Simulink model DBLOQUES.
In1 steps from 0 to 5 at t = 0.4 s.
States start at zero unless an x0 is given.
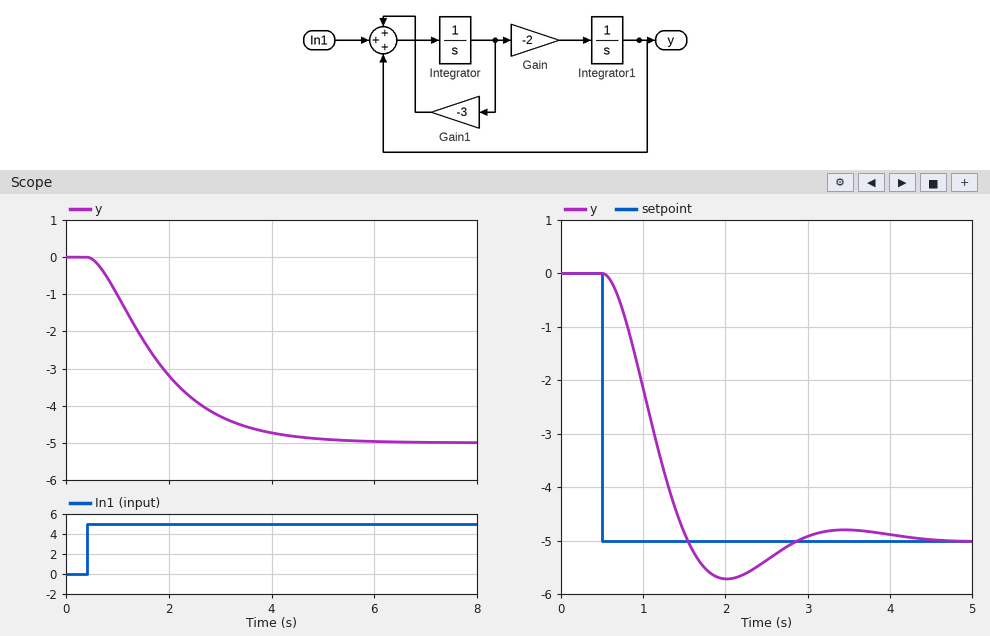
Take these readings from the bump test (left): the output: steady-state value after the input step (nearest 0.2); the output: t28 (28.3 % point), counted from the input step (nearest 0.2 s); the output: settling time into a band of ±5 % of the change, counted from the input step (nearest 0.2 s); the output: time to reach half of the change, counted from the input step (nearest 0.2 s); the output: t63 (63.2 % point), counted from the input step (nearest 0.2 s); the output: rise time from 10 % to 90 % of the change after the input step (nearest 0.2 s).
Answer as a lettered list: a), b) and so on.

a) -5.0
b) 0.8 s
c) 3.6 s
d) 1.2 s
e) 1.6 s
f) 2.6 s
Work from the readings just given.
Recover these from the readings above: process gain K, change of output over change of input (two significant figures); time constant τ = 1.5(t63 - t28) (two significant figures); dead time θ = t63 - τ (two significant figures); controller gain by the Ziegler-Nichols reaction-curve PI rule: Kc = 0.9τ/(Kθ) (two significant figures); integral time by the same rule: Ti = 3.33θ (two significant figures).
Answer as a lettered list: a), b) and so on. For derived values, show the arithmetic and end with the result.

a) (-5 - 0) / 5 = -1.0
b) 1.5 × (1.6 - 0.8) = 1.2 s
c) 1.6 - 1.2 = 0.40 s
d) 0.9 × 1.2 / (-1 × 0.4) = -2.7
e) 3.33 × 0.4 = 1.3 s
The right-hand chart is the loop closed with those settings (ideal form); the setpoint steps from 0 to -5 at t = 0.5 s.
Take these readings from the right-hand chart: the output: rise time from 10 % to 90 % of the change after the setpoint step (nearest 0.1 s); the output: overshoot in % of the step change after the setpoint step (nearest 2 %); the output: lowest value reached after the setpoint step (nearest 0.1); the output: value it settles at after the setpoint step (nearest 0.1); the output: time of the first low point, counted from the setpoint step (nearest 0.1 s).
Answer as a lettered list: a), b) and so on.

a) 0.7 s
b) 14 %
c) -5.7
d) -5.0
e) 1.5 s
